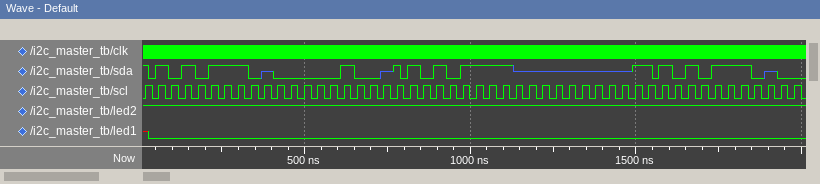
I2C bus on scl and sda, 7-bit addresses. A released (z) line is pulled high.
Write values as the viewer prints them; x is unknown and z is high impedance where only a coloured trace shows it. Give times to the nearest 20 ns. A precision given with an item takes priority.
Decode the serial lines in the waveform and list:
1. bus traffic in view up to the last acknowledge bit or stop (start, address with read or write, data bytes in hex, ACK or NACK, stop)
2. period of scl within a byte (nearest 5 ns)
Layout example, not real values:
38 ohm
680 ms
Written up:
start, address 57 write NACK, 04 NACK, repeated start, address 57 read NACK, FF NACK, repeated start, address 57 write NACK
40 ns
